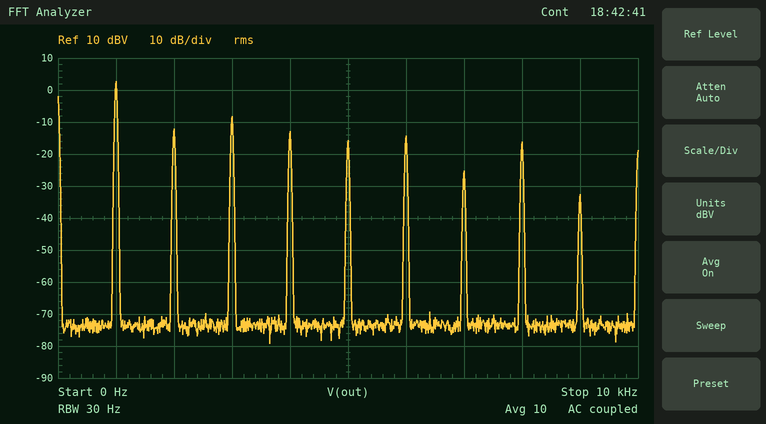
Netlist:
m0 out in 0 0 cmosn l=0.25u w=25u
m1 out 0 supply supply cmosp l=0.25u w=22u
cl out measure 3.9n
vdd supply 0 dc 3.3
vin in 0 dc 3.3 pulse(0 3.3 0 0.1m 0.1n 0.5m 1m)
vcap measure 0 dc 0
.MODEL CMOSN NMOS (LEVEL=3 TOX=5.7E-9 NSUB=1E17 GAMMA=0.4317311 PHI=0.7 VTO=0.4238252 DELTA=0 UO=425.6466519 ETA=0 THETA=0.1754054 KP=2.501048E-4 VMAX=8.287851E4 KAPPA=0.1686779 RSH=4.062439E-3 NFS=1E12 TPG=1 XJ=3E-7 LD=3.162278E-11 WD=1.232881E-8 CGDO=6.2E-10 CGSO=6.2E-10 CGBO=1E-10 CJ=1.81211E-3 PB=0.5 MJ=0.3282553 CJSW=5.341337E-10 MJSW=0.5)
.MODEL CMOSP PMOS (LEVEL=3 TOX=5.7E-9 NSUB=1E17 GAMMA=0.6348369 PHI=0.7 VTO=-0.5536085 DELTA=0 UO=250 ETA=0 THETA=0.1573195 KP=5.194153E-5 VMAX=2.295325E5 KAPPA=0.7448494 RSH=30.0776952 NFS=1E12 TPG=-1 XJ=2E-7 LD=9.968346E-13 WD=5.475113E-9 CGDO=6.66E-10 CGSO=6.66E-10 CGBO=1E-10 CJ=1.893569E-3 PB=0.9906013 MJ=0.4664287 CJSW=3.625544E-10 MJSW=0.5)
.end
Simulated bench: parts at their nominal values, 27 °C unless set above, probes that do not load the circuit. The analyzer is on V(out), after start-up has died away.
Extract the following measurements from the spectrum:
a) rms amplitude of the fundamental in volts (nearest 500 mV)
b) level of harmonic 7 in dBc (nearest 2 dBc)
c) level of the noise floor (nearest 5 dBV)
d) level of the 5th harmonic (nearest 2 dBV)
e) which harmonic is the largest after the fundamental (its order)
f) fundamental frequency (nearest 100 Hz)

1.5 V
-28 dBc
-75 dBV
-16 dBV
3
1.0 kHz
